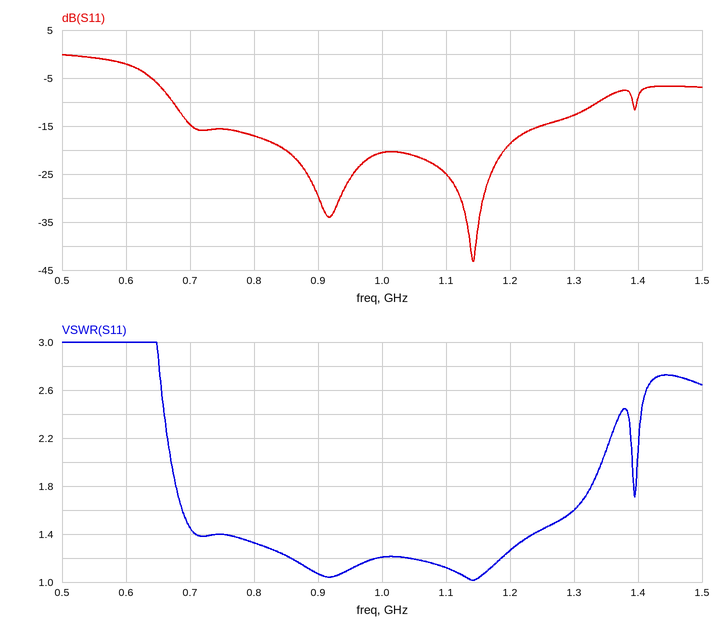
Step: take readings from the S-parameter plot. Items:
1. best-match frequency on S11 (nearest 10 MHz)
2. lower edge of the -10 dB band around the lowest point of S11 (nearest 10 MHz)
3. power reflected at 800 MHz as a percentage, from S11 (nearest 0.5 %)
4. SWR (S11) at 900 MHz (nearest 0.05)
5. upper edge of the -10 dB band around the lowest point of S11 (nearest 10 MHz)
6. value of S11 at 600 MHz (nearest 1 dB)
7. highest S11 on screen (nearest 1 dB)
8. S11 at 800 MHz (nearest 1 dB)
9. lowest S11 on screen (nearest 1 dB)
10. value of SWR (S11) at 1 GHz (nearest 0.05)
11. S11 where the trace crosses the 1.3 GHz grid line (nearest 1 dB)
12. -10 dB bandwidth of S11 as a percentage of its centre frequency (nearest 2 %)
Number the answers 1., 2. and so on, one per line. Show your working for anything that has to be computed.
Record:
1. 1.14 GHz
2. 670 MHz
3. 10^(-17/10) ≈ 2.0 %
4. 1.05
5. 1.34 GHz
6. -2 dB
7. 0 dB
8. -17 dB
9. -43 dB
10. 1.20
11. -13 dB
12. 670 MHz / 1.005 GHz ≈ 66.7 %, so 66 % to the nearest 2 %
